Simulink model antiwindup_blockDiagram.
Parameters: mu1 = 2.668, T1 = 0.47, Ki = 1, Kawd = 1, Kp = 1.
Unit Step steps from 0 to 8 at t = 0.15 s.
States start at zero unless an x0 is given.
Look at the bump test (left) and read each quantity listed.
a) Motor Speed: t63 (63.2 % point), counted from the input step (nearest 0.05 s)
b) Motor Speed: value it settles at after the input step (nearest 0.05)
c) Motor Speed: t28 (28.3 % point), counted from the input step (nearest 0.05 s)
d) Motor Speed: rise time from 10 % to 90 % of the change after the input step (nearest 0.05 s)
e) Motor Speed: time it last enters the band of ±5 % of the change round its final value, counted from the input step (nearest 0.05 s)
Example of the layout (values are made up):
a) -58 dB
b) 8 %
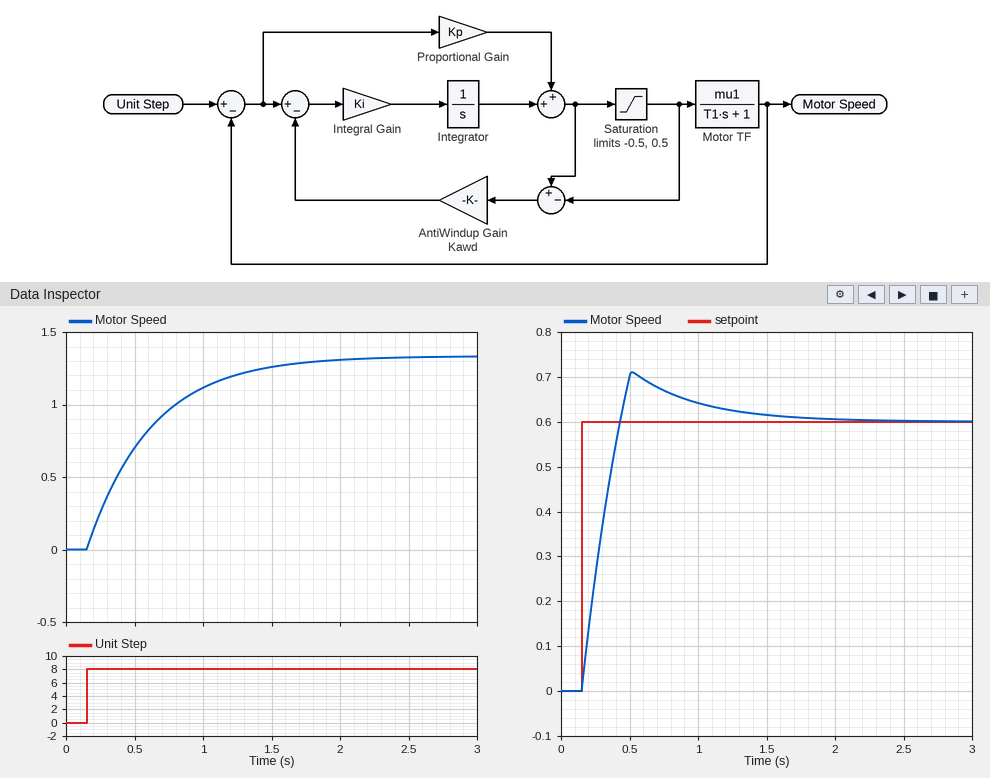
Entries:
a) 0.45 s
b) 1.35
c) 0.15 s
d) 1.05 s
e) 1.40 s
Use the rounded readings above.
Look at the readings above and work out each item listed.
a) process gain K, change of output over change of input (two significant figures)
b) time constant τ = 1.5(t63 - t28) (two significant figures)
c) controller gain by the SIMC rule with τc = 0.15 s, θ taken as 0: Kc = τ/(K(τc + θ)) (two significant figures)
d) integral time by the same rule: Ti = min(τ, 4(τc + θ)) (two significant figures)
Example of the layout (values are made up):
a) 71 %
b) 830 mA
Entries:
a) 0.17
b) 0.45 s
c) 18
d) 0.45 s
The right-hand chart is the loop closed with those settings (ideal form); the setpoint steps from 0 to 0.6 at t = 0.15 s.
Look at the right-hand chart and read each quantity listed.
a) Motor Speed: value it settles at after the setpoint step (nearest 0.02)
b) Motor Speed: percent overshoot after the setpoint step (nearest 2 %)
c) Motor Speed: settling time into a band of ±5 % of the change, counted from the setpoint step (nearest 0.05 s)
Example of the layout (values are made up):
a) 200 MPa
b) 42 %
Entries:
a) 0.60
b) 18 %
c) 1.00 s
